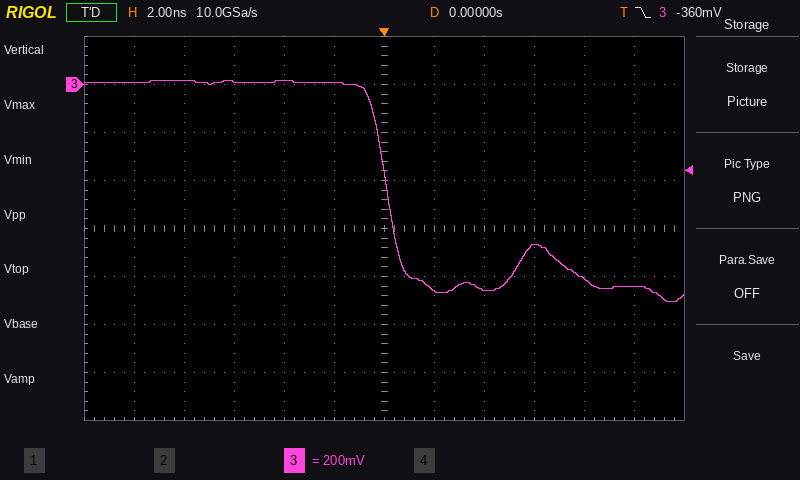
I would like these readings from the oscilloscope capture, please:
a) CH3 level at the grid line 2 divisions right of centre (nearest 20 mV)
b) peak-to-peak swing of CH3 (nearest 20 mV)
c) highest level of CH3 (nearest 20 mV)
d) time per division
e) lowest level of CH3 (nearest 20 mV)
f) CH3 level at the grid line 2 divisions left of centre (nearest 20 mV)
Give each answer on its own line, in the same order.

-860 mV
920 mV
20 mV
2 ns
-900 mV
20 mV
